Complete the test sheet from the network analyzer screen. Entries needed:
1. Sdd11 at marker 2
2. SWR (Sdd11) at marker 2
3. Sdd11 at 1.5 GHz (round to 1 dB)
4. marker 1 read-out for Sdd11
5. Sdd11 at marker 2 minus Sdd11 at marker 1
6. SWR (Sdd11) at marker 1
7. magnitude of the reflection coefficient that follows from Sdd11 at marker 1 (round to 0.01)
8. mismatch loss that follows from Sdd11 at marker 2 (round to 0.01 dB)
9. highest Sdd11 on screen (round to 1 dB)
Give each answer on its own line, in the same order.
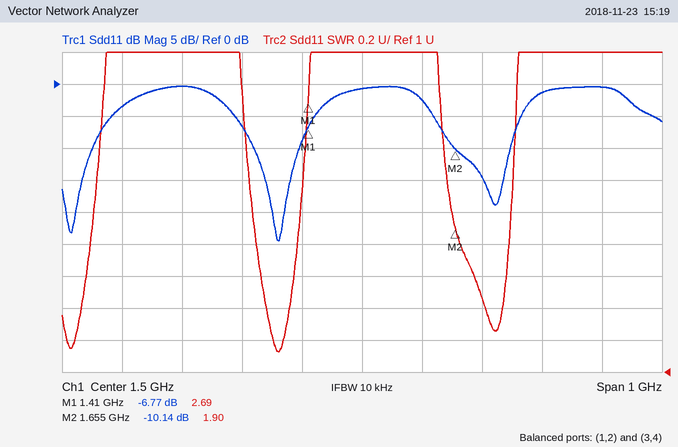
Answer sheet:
-10.14 dB
1.90
-1 dB
-6.77 dB
-3.37 dB
2.69
0.46
0.44 dB
0 dB
